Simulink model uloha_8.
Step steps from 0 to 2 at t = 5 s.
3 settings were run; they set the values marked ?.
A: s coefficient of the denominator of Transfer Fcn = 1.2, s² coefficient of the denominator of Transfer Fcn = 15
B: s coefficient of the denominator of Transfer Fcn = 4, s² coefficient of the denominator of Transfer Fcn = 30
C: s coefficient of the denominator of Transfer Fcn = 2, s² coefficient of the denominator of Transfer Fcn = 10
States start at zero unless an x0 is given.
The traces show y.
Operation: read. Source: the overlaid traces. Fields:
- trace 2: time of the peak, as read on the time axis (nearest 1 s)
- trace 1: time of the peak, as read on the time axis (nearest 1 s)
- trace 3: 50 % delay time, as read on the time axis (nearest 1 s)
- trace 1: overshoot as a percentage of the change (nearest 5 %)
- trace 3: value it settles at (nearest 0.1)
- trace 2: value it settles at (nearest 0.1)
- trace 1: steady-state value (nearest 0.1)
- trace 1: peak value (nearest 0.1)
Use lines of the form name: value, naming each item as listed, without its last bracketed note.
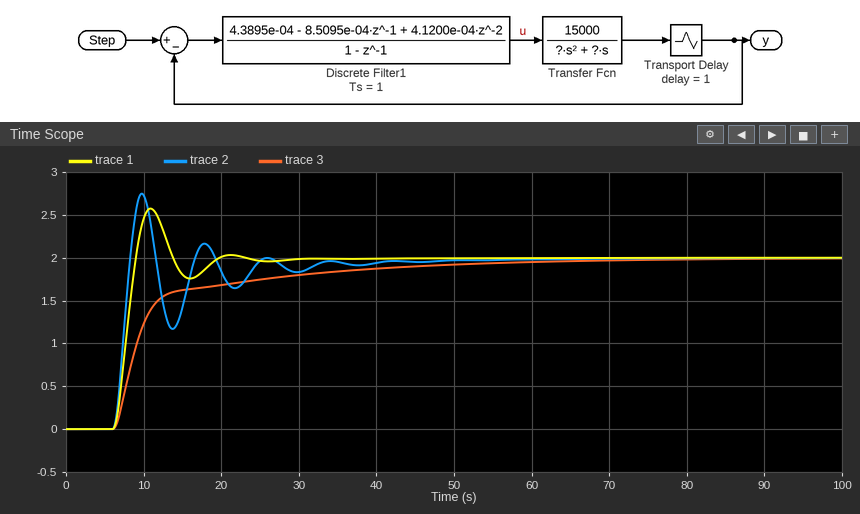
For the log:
trace 2: time of the peak, as read on the time axis: 10 s
trace 1: time of the peak, as read on the time axis: 11 s
trace 3: 50 % delay time, as read on the time axis: 9 s
trace 1: overshoot as a percentage of the change: 30 %
trace 3: value it settles at: 2.0
trace 2: value it settles at: 2.0
trace 1: steady-state value: 2.0
trace 1: peak value: 2.6
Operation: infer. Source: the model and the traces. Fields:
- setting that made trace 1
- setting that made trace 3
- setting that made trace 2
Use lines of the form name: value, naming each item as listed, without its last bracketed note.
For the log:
setting that made trace 1: A
setting that made trace 3: B
setting that made trace 2: C
